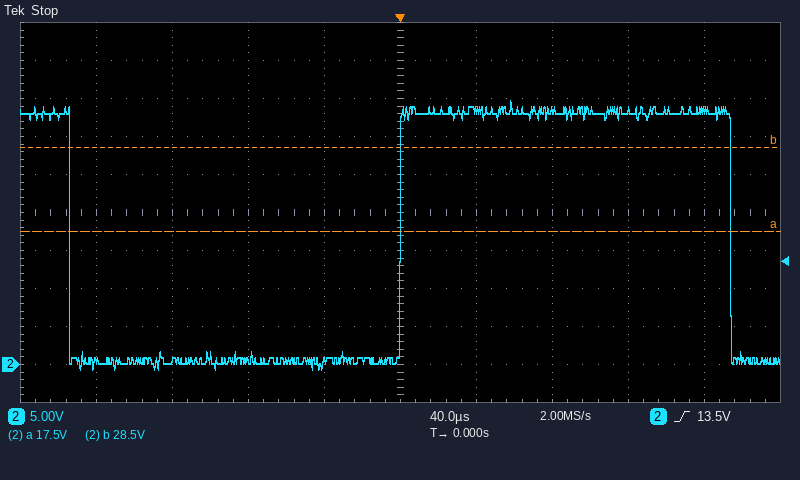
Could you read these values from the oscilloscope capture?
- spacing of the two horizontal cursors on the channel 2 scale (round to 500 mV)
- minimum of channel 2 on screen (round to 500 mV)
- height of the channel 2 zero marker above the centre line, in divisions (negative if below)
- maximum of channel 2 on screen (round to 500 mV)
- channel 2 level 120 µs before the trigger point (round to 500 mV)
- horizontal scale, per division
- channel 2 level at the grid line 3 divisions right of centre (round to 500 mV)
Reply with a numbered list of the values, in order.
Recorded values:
1. 11.0 V
2. -500 mV
3. -4.0 div
4. 34.5 V
5. 500 mV
6. 40 µs
7. 33.5 V
